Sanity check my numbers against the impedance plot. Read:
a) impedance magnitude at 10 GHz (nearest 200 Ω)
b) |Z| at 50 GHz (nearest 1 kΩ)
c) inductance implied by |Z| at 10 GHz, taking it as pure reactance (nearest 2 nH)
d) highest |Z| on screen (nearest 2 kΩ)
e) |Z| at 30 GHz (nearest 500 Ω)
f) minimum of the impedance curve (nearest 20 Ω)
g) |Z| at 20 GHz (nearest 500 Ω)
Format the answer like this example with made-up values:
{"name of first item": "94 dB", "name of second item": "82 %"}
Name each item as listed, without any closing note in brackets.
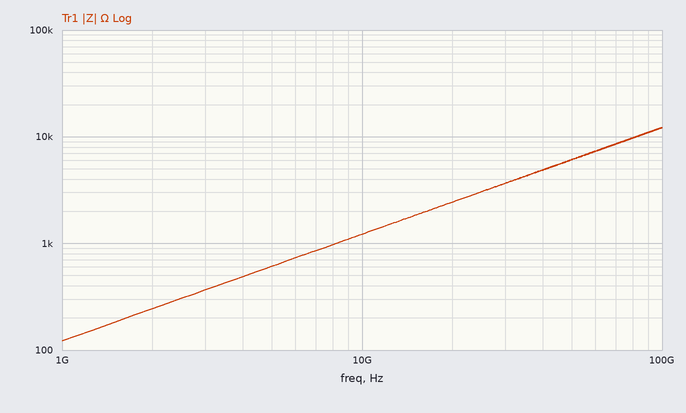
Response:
{"impedance magnitude at 10 GHz": "1.2 kΩ", "|Z| at 50 GHz": "6 kΩ", "inductance implied by |Z| at 10 GHz, taking it as pure reactance": "20 nH", "highest |Z| on screen": "12 kΩ", "|Z| at 30 GHz": "3.5 kΩ", "minimum of the impedance curve": "120 Ω", "|Z| at 20 GHz": "2.5 kΩ"}
